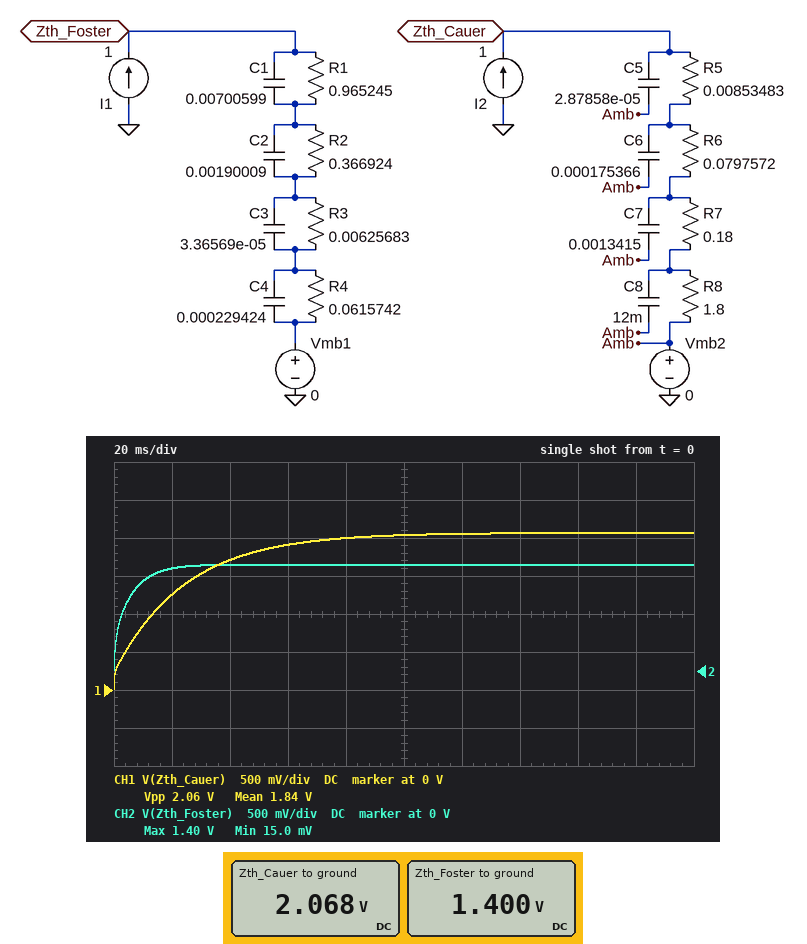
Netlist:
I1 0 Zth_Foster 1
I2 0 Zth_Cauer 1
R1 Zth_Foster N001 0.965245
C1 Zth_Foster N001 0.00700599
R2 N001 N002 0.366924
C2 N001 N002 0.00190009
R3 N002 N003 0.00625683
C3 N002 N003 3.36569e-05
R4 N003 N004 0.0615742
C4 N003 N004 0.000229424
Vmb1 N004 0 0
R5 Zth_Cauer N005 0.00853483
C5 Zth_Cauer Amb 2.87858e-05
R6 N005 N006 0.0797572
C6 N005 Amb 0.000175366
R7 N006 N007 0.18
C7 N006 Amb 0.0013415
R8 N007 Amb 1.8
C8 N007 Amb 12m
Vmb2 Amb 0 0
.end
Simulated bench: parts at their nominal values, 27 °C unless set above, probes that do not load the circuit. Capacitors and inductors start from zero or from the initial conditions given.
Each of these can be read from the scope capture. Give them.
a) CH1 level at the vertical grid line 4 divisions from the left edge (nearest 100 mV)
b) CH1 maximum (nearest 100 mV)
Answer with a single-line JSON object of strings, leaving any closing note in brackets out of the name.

{"CH1 level at the vertical grid line 4 divisions from the left edge": "2.0 V", "CH1 maximum": "2.1 V"}
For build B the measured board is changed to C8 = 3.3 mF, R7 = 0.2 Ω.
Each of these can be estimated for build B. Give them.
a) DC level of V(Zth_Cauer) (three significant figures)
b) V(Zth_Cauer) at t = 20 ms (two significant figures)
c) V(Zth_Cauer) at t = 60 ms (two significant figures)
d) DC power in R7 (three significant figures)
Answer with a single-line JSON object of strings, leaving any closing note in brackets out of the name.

{"DC level of V(Zth_Cauer)": "2.09 V", "V(Zth_Cauer) at t = 20 ms": "1.9 V", "V(Zth_Cauer) at t = 60 ms": "2.1 V", "DC power in R7": "200 mW"}
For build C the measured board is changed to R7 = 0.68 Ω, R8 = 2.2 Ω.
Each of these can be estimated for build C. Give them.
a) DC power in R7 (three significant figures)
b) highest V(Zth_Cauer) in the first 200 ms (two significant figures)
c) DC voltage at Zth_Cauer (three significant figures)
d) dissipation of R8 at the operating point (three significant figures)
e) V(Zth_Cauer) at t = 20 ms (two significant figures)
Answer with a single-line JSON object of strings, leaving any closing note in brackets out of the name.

{"DC power in R7": "680 mW", "highest V(Zth_Cauer) in the first 200 ms": "3.0 V", "DC voltage at Zth_Cauer": "2.97 V", "dissipation of R8 at the operating point": "2.20 W", "V(Zth_Cauer) at t = 20 ms": "1.8 V"}
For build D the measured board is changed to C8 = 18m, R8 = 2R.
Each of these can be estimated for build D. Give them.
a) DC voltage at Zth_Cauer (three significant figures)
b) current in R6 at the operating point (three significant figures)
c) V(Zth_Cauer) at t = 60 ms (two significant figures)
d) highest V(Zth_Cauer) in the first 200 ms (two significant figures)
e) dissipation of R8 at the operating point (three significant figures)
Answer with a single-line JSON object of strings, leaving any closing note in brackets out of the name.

{"DC voltage at Zth_Cauer": "2.27 V", "current in R6 at the operating point": "1.00 A", "V(Zth_Cauer) at t = 60 ms": "1.8 V", "highest V(Zth_Cauer) in the first 200 ms": "2.3 V", "dissipation of R8 at the operating point": "2.00 W"}
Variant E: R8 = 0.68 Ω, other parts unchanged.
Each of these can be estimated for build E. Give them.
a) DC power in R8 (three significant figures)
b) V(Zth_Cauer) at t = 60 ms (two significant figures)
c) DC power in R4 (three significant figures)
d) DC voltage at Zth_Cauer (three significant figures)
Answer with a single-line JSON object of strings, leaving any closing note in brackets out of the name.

{"DC power in R8": "680 mW", "V(Zth_Cauer) at t = 60 ms": "950 mV", "DC power in R4": "61.6 mW", "DC voltage at Zth_Cauer": "948 mV"}
